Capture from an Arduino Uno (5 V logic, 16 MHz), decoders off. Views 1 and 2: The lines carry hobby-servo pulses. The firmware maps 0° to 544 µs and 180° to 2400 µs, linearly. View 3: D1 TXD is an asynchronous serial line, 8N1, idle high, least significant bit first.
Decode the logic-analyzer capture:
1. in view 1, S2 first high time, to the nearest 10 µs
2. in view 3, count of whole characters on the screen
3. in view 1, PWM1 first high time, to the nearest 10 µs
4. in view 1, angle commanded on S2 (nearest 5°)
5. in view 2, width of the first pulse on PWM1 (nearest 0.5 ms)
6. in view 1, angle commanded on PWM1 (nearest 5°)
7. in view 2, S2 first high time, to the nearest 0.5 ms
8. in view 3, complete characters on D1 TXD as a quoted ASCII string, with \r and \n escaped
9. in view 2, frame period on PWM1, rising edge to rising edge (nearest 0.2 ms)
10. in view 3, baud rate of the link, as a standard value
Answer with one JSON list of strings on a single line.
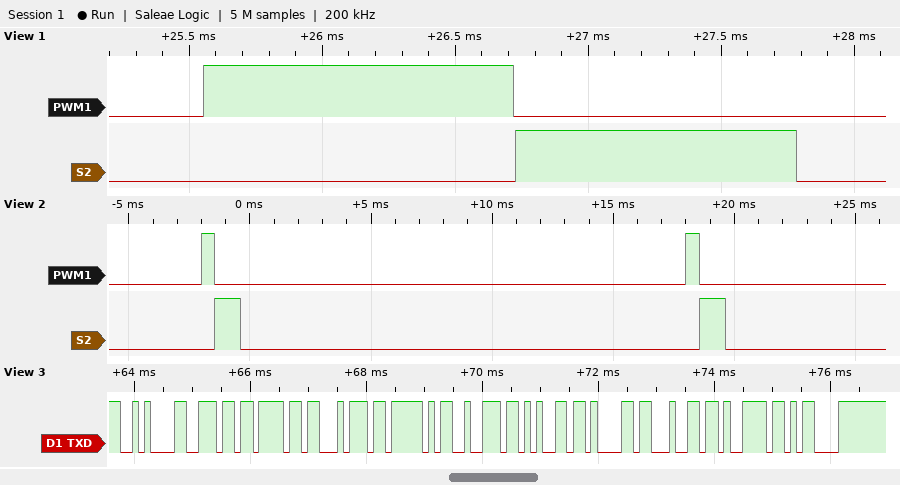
["1060 µs", "11", "1160 µs", "50°", "0.5 ms", "60°", "1.0 ms", "\"\\nnot_ready\\r\"", "20.0 ms", "9600 baud"]
